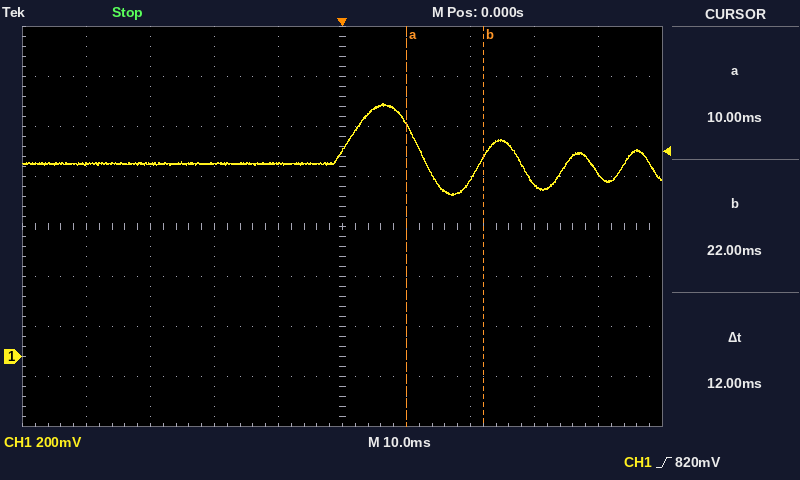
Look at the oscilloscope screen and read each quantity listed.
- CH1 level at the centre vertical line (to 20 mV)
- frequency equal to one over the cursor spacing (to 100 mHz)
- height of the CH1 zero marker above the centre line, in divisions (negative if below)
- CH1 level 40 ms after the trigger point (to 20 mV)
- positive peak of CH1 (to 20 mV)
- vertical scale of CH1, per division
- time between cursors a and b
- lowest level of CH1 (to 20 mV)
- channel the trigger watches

820 mV
83.3 Hz
-2.6 div
740 mV
1.02 V
200 mV
12 ms
640 mV
CH1
